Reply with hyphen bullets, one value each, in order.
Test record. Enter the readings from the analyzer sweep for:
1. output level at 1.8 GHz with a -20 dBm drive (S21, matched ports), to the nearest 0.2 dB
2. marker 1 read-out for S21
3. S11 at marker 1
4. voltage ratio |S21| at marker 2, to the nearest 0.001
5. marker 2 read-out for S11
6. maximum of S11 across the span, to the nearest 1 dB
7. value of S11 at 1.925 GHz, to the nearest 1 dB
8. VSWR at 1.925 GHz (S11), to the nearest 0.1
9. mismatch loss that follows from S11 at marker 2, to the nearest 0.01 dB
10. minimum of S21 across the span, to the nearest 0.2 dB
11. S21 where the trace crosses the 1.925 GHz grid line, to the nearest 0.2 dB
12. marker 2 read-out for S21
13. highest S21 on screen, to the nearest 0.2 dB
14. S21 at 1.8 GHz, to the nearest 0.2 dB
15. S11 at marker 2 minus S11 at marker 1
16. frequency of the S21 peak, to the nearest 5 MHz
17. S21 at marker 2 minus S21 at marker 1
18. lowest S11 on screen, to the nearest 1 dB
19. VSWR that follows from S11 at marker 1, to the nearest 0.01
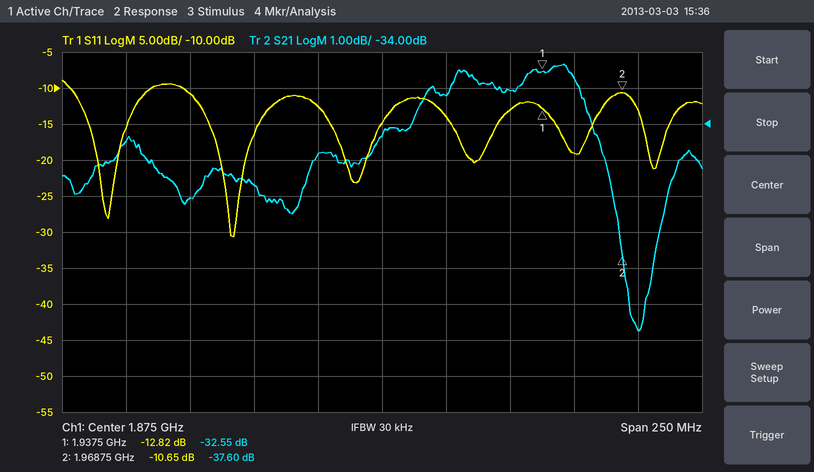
- -56.0 dBm
- -32.55 dB
- -12.82 dB
- 0.013
- -10.65 dB
- -9 dB
- -13 dB
- 1.6
- 0.39 dB
- -39.8 dB
- -33.0 dB
- -37.60 dB
- -32.4 dB
- -36.0 dB
- 2.17 dB
- 1.945 GHz
- -5.05 dB
- -31 dB
- 1.59
